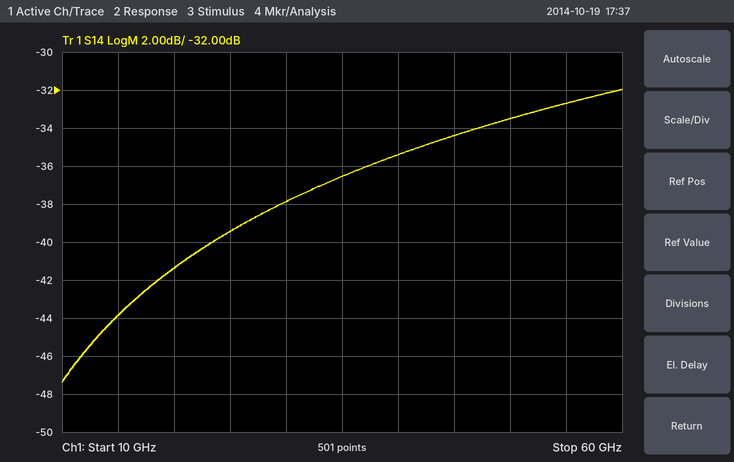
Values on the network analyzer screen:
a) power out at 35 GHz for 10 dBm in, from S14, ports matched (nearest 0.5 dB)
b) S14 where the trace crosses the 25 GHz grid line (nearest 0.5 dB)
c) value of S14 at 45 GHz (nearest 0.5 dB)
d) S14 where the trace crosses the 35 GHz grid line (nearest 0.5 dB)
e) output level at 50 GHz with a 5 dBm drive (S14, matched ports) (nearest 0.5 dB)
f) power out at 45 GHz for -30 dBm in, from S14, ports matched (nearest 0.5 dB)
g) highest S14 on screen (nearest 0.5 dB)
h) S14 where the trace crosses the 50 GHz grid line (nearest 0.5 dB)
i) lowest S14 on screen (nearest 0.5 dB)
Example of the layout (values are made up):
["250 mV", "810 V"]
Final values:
["-26.5 dBm", "-39.5 dB", "-34.5 dB", "-36.5 dB", "-28.5 dBm", "-64.5 dBm", "-32.0 dB", "-33.5 dB", "-47.5 dB"]
